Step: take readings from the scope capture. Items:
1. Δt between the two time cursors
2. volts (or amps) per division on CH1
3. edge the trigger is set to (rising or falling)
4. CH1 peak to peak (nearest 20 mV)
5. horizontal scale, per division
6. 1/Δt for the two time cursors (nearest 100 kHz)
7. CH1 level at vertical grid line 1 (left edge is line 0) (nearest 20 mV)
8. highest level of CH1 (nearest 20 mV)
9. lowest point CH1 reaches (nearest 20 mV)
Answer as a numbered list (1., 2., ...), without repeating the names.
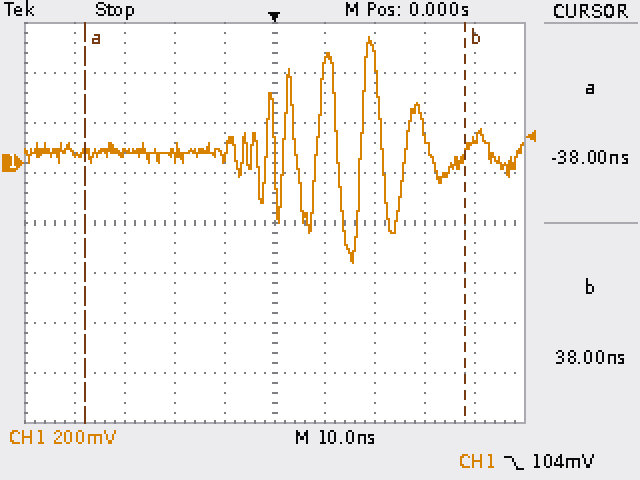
1. 76 ns
2. 200 mV
3. falling
4. 900 mV
5. 10 ns
6. 13.2 MHz
7. 40 mV
8. 500 mV
9. -400 mV
